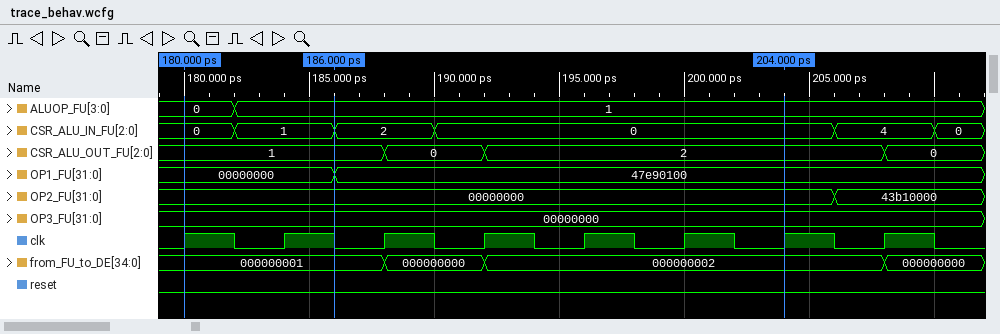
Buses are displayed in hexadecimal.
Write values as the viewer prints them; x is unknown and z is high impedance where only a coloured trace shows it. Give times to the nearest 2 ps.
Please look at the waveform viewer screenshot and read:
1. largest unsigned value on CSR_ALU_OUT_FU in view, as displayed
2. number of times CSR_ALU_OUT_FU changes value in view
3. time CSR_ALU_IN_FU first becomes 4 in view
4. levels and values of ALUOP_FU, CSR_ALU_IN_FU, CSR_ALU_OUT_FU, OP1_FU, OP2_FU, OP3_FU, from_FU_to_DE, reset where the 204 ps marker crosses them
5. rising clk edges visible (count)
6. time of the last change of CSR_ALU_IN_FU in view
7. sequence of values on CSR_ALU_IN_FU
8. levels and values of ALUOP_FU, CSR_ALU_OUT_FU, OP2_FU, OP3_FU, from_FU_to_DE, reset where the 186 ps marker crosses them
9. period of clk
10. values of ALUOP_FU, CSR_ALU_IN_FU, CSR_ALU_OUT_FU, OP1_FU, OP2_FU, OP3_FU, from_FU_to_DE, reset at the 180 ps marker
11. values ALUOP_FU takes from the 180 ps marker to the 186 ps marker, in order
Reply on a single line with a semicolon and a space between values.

2; 3; 206 ps; ALUOP_FU=1, CSR_ALU_IN_FU=0, CSR_ALU_OUT_FU=2, OP1_FU=47e90100, OP2_FU=00000000, OP3_FU=00000000, from_FU_to_DE=000000002, reset=0; 8; 210 ps; 0, 1, 2, 0, 4, 0; ALUOP_FU=1, CSR_ALU_OUT_FU=1, OP2_FU=00000000, OP3_FU=00000000, from_FU_to_DE=000000001, reset=0; 4 ps; ALUOP_FU=0, CSR_ALU_IN_FU=0, CSR_ALU_OUT_FU=1, OP1_FU=00000000, OP2_FU=00000000, OP3_FU=00000000, from_FU_to_DE=000000001, reset=0; 0, 1
